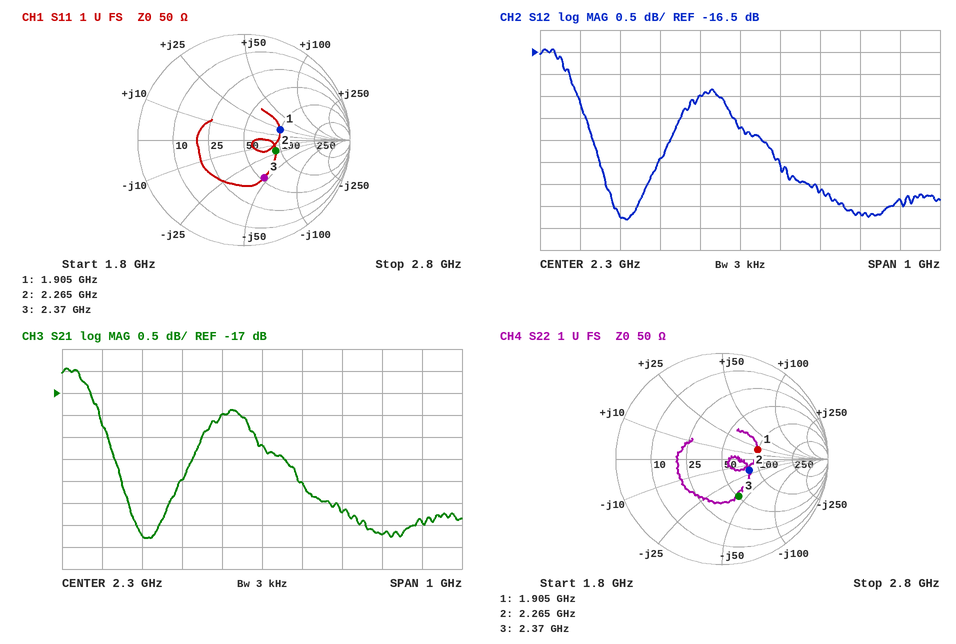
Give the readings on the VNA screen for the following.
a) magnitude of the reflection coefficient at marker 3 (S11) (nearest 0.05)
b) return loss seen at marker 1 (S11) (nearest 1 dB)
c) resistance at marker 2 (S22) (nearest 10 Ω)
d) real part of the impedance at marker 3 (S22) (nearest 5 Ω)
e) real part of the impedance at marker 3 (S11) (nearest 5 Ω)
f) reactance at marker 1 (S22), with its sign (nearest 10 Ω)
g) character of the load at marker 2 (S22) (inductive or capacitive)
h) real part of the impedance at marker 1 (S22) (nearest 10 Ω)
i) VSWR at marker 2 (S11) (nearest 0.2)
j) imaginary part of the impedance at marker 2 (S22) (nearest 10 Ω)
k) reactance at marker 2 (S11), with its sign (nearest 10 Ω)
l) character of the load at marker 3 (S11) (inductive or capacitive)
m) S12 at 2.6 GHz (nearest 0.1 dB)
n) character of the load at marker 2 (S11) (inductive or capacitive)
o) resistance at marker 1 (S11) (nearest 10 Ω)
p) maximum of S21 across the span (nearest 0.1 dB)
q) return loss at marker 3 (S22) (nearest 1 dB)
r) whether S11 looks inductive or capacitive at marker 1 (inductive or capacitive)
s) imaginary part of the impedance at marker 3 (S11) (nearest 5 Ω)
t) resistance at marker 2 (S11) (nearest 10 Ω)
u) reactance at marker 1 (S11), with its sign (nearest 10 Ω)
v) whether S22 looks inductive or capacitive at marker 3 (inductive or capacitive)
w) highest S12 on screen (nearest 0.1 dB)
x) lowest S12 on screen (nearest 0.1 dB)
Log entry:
0.40
9 dB
80 Ω
50 Ω
55 Ω
+20 Ω
capacitive
100 Ω
2.0
-20 Ω
-20 Ω
capacitive
-20.2 dB
capacitive
100 Ω
-16.4 dB
8 dB
inductive
-45 Ω
90 Ω
+20 Ω
capacitive
-16.4 dB
-20.3 dB
